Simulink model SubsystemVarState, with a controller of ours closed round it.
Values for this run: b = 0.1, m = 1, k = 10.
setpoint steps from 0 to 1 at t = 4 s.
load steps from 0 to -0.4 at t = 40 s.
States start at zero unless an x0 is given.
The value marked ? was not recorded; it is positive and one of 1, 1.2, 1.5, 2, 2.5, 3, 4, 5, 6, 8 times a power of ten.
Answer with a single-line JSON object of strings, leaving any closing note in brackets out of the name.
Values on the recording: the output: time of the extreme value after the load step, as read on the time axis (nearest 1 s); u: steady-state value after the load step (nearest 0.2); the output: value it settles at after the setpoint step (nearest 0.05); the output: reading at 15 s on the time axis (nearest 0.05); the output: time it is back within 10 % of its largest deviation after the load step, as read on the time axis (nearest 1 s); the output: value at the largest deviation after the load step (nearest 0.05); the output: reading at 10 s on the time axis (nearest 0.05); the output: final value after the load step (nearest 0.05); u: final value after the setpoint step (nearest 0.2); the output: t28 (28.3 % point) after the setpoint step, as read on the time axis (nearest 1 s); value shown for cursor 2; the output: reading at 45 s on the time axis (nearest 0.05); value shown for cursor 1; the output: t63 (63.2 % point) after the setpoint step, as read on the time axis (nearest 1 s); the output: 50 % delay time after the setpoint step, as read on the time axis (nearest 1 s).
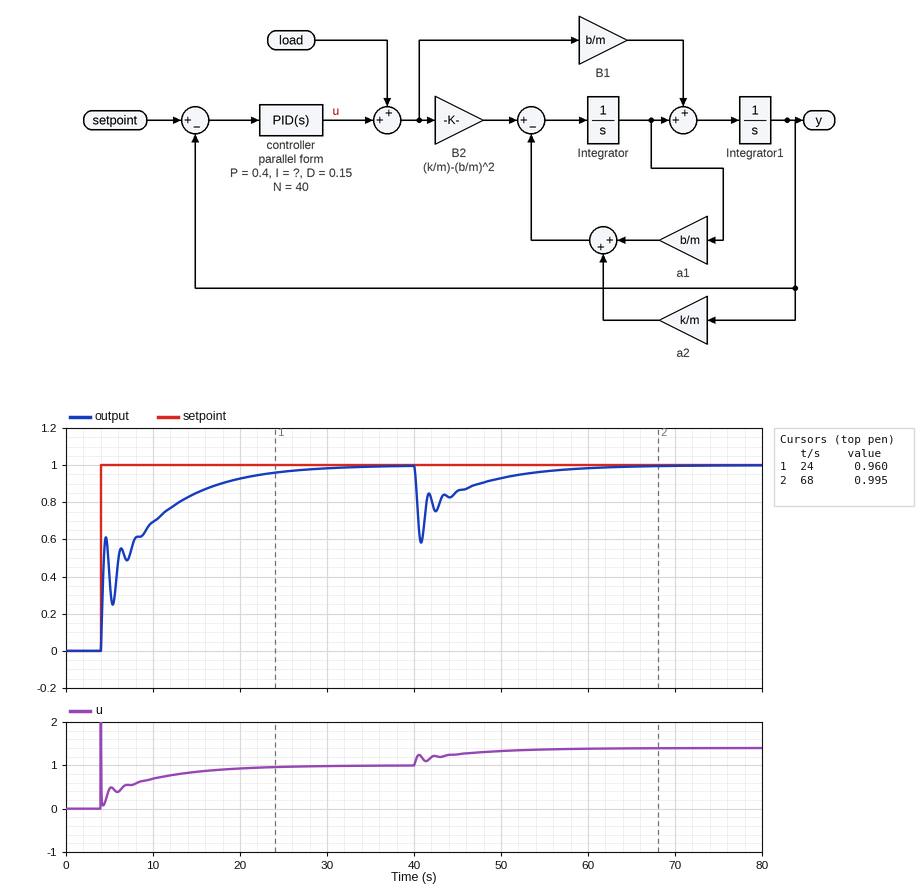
{"the output: time of the extreme value after the load step, as read on the time axis": "41 s", "u: steady-state value after the load step": "1.4", "the output: value it settles at after the setpoint step": "1.00", "the output: reading at 15 s on the time axis": "0.85", "the output: time it is back within 10 % of its largest deviation after the load step, as read on the time axis": "54 s", "the output: value at the largest deviation after the load step": "0.60", "the output: reading at 10 s on the time axis": "0.70", "the output: final value after the load step": "1.00", "u: final value after the setpoint step": "1.0", "the output: t28 (28.3 % point) after the setpoint step, as read on the time axis": "4 s", "value shown for cursor 2": "0.995", "the output: reading at 45 s on the time axis": "0.85", "value shown for cursor 1": "0.960", "the output: t63 (63.2 % point) after the setpoint step, as read on the time axis": "9 s", "the output: 50 % delay time after the setpoint step, as read on the time axis": "4 s"}
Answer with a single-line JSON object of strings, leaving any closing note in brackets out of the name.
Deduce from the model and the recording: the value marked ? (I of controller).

{"the value marked ?": "0.2"}
